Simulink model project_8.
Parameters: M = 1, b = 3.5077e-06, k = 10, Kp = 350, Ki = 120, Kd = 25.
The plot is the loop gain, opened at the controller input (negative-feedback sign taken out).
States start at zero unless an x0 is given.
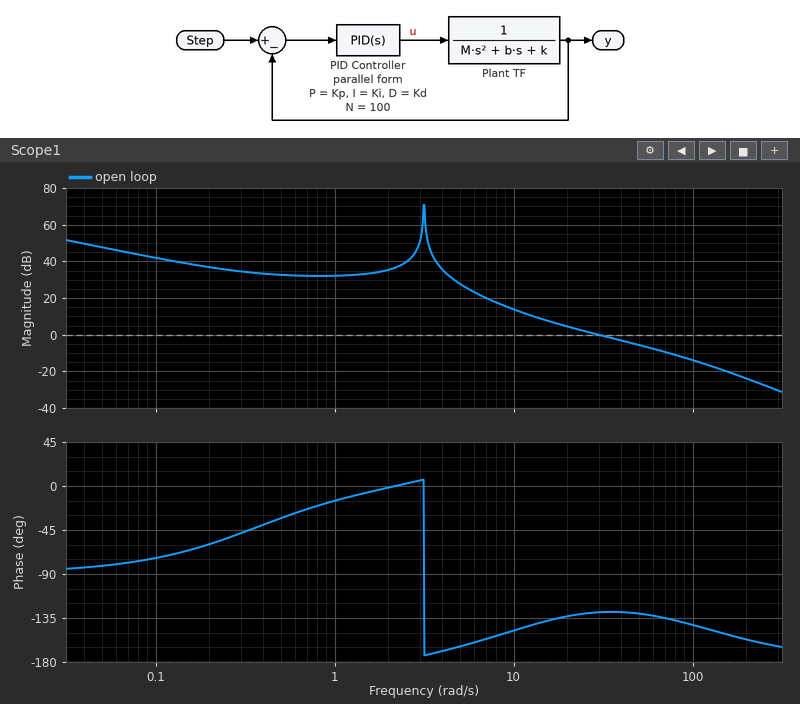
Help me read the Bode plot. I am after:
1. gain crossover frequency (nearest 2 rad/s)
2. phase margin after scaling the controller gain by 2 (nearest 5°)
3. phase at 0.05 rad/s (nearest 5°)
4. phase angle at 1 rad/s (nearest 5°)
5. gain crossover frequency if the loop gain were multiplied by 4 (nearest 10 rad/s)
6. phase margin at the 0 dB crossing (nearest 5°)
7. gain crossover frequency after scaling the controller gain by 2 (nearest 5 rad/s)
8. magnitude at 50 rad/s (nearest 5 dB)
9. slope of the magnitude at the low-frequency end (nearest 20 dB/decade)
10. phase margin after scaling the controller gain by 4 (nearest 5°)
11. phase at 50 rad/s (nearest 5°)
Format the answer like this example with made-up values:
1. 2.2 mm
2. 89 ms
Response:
1. 30 rad/s
2. 50°
3. -80°
4. -15°
5. 90 rad/s
6. 50°
7. 50 rad/s
8. -5 dB
9. -20 dB/decade
10. 40°
11. -130°
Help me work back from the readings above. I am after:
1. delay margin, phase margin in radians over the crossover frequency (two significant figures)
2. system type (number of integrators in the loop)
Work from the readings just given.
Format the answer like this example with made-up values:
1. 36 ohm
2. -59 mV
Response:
1. 0.029 s
2. 1
